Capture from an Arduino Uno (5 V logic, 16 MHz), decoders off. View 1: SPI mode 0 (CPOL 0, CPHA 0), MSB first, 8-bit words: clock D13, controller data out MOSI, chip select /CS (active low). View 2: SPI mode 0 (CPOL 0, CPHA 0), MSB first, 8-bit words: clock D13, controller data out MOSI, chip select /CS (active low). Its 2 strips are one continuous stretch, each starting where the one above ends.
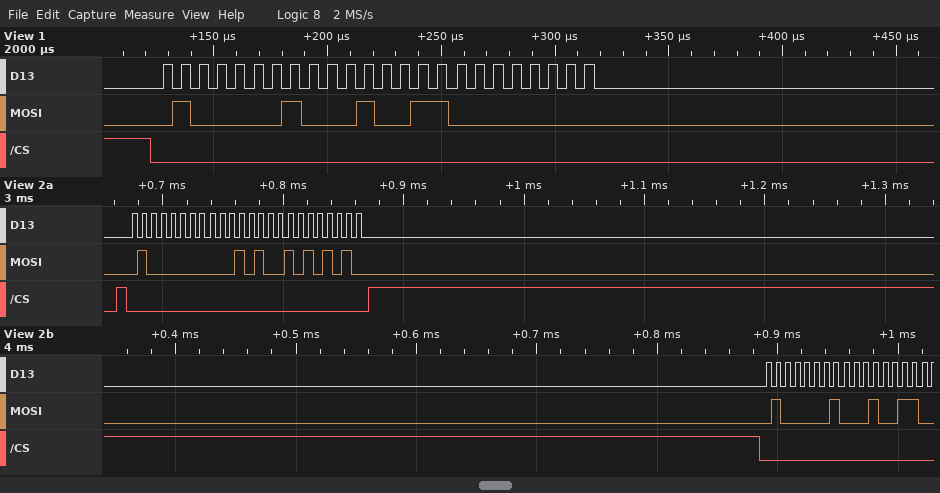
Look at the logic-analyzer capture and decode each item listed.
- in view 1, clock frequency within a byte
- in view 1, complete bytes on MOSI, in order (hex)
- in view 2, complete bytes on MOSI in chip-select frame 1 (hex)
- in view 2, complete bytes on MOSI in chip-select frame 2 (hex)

125 kHz
0x41 0x13 0x00
40 14 AA
41 13
